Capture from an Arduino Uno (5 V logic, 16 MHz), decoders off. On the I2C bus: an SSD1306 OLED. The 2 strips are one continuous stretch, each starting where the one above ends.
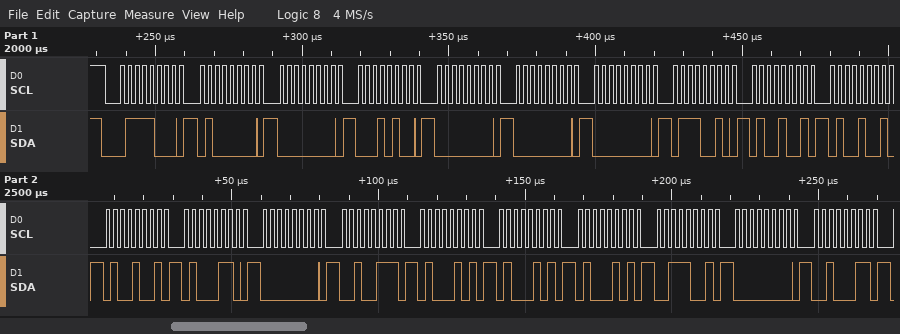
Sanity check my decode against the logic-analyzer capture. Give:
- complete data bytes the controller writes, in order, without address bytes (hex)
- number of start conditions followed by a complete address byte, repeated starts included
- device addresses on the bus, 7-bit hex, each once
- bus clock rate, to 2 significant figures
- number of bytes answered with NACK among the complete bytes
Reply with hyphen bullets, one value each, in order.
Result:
- 40 00 14 00 00 00 72 49 49 49 46 00 27 45 45 45 39 00 23
- 1
- 0x3C
- 400 kHz
- 0
